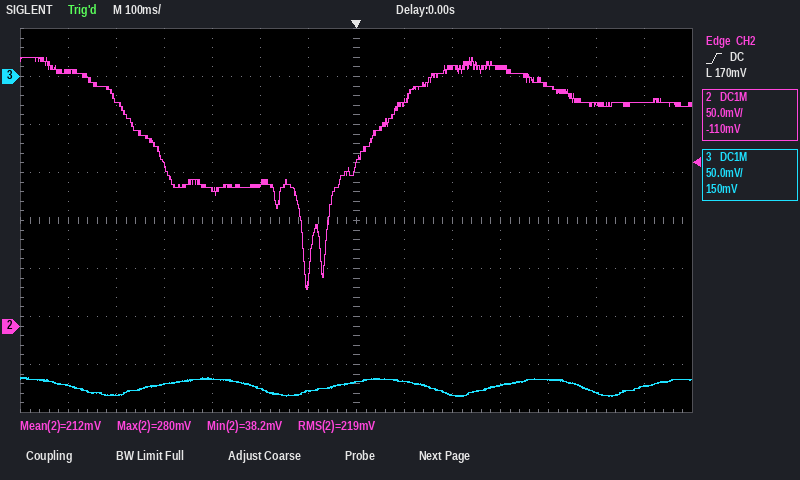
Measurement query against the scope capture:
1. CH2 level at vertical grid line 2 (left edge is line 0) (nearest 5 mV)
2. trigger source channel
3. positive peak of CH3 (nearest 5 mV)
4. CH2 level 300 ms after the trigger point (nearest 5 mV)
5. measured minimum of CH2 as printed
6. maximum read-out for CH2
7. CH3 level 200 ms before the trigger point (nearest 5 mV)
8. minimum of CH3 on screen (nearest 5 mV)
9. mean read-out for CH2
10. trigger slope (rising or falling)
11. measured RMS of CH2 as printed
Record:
235 mV
CH2
-315 mV
270 mV
38.2 mV
280 mV
-325 mV
-335 mV
212 mV
rising
219 mV
